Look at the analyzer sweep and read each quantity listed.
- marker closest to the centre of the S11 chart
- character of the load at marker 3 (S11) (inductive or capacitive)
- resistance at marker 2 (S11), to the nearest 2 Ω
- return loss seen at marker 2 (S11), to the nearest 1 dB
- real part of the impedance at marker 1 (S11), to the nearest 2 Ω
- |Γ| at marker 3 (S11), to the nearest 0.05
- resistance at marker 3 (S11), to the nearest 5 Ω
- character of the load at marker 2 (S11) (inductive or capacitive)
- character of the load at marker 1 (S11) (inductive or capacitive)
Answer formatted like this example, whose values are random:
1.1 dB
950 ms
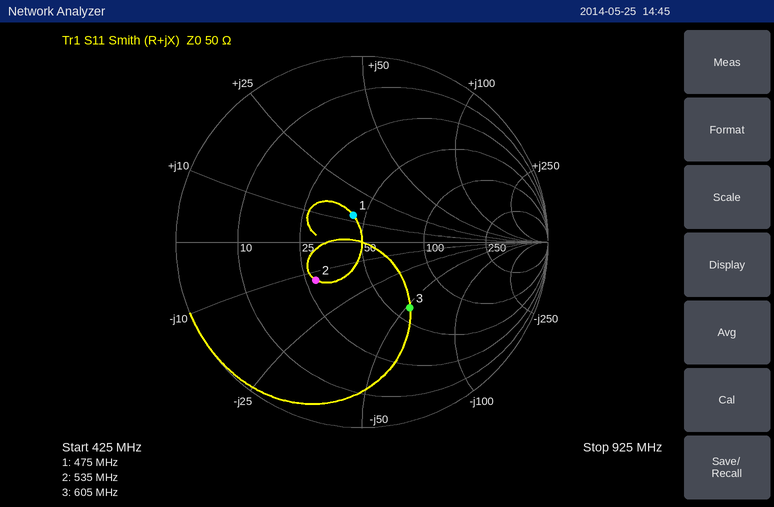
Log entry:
marker 1
capacitive
28 Ω
10 dB
44 Ω
0.45
60 Ω
capacitive
inductive
